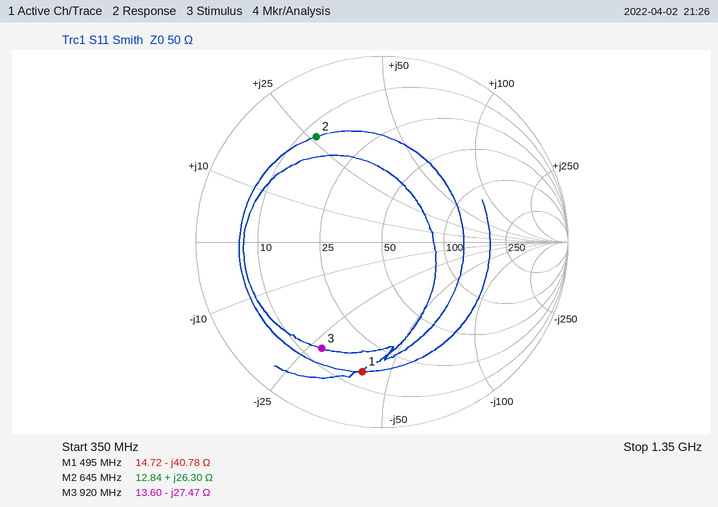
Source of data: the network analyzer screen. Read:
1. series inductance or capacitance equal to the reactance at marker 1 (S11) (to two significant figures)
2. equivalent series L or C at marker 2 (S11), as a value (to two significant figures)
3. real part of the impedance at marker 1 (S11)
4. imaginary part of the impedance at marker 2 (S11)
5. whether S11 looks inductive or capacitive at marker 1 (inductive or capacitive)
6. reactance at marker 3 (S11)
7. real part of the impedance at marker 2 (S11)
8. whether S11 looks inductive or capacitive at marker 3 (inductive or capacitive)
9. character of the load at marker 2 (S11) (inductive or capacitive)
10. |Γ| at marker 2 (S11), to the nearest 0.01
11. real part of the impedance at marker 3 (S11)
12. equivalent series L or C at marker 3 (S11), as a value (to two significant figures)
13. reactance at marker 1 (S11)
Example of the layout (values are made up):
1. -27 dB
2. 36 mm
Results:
1. 7.9 pF
2. 6.5 nH
3. 14.72 Ω
4. +26.30 Ω
5. capacitive
6. -27.47 Ω
7. 12.84 Ω
8. capacitive
9. inductive
10. 0.67
11. 13.60 Ω
12. 6.3 pF
13. -40.78 Ω
